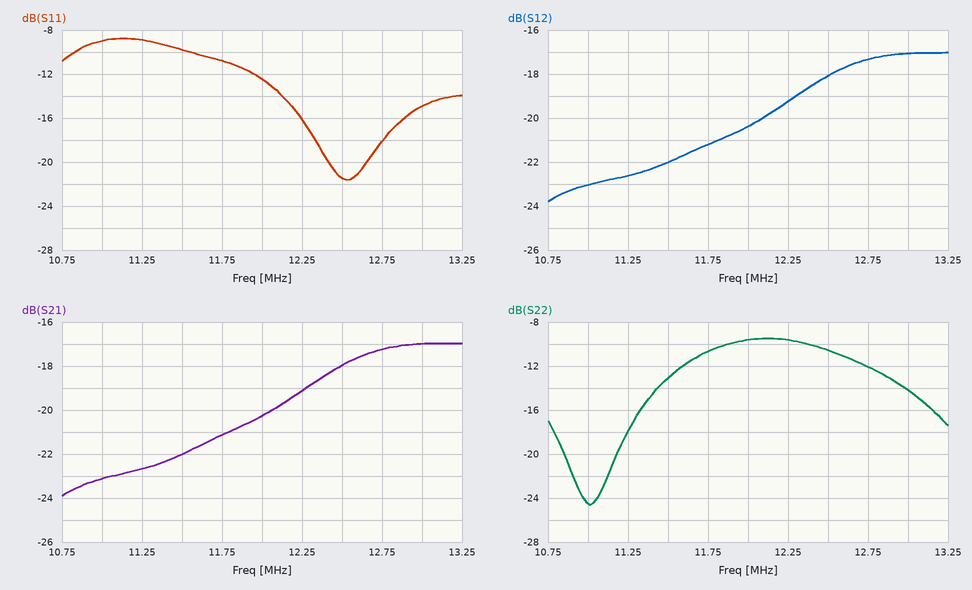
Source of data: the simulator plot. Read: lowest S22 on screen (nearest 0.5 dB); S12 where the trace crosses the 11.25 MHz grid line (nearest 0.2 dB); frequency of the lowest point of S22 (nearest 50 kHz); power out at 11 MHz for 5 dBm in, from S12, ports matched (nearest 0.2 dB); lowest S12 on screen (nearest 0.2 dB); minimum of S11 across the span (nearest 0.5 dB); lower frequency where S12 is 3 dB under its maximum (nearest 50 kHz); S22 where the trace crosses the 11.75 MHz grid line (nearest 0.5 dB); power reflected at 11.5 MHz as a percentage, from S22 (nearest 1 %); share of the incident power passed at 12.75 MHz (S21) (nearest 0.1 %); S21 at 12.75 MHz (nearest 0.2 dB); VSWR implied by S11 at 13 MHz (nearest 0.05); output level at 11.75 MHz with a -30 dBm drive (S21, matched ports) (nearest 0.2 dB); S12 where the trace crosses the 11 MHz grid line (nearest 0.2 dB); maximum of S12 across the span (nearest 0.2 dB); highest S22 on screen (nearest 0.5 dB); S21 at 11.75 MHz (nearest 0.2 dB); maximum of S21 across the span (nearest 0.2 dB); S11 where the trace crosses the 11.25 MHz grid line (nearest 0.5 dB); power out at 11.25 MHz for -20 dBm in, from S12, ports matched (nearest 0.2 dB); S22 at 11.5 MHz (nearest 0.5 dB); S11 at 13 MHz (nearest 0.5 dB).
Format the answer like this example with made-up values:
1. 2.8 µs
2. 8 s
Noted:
1. -24.5 dB
2. -22.6 dB
3. 11.00 MHz
4. -18.0 dBm
5. -23.8 dB
6. -21.5 dB
7. 12.10 MHz
8. -10.5 dB
9. 5 %
10. 1.9 %
11. -17.2 dB
12. 1.45
13. -51.2 dBm
14. -23.0 dB
15. -17.0 dB
16. -9.5 dB
17. -21.2 dB
18. -17.0 dB
19. -9.0 dB
20. -42.6 dBm
21. -13.0 dB
22. -15.0 dB
